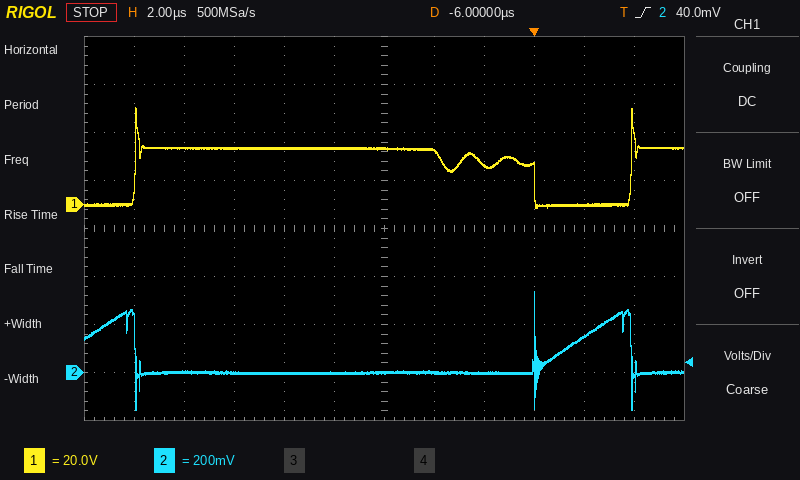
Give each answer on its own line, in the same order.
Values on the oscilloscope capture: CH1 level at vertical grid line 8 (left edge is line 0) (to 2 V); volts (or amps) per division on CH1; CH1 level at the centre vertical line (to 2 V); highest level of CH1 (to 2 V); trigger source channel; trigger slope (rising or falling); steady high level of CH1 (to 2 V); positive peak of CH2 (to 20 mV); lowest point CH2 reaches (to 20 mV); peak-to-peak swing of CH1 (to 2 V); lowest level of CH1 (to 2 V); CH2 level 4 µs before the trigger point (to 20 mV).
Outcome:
16 V
20 V
24 V
40 V
CH2
rising
24 V
340 mV
-160 mV
42 V
-2 V
0 mV
